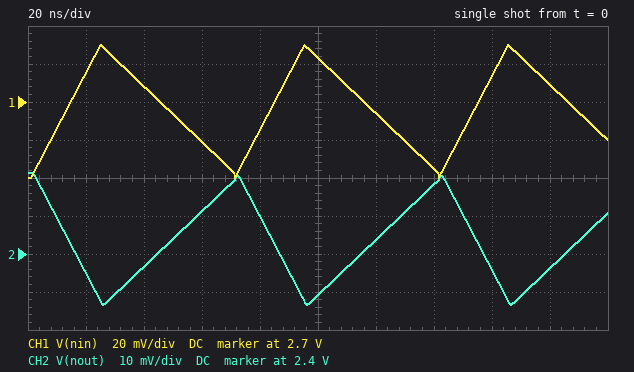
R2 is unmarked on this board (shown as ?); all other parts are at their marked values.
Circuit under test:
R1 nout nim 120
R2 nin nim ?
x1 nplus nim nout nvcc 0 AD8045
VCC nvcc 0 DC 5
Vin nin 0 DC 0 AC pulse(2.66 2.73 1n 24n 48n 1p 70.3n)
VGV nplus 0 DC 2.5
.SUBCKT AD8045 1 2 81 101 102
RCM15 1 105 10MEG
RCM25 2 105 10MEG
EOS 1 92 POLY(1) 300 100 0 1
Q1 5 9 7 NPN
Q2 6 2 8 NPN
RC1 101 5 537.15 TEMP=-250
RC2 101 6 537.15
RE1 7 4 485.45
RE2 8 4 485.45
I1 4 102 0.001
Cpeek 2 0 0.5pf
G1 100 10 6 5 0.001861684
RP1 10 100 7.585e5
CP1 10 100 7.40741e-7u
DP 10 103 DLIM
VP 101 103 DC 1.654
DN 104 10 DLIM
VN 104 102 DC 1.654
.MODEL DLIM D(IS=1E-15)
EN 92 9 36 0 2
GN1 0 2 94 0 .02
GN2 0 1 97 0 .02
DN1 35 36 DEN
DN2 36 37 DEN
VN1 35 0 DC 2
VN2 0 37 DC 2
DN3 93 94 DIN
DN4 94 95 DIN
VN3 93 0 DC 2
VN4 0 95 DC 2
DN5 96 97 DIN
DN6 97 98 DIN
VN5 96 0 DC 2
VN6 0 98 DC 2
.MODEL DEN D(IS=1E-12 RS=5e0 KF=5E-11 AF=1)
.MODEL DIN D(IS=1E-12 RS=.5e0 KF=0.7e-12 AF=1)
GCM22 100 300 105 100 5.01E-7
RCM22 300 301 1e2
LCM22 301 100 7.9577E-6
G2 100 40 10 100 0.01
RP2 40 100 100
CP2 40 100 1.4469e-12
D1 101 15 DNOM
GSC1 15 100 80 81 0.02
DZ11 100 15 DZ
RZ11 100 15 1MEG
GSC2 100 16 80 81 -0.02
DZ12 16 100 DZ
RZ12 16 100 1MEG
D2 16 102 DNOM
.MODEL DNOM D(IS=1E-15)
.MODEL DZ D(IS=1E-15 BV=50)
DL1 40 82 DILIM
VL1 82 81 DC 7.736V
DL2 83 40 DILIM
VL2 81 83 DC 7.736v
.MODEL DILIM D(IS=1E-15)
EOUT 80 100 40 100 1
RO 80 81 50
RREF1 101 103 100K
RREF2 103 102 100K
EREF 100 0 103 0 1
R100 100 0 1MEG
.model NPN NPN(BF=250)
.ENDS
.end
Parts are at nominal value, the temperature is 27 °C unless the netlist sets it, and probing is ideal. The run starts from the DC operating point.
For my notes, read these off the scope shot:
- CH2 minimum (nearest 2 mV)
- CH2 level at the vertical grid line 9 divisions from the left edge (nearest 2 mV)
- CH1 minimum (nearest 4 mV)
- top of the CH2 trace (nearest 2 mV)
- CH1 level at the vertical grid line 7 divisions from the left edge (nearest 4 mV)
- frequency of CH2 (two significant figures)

2.386 V
2.396 V
2.660 V
2.422 V
2.664 V
14 MHz
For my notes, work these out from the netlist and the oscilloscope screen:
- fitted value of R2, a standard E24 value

240 Ω
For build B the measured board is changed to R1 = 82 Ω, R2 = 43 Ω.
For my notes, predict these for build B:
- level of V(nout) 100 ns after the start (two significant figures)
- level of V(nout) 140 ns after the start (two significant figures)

2.1 V
2.2 V
